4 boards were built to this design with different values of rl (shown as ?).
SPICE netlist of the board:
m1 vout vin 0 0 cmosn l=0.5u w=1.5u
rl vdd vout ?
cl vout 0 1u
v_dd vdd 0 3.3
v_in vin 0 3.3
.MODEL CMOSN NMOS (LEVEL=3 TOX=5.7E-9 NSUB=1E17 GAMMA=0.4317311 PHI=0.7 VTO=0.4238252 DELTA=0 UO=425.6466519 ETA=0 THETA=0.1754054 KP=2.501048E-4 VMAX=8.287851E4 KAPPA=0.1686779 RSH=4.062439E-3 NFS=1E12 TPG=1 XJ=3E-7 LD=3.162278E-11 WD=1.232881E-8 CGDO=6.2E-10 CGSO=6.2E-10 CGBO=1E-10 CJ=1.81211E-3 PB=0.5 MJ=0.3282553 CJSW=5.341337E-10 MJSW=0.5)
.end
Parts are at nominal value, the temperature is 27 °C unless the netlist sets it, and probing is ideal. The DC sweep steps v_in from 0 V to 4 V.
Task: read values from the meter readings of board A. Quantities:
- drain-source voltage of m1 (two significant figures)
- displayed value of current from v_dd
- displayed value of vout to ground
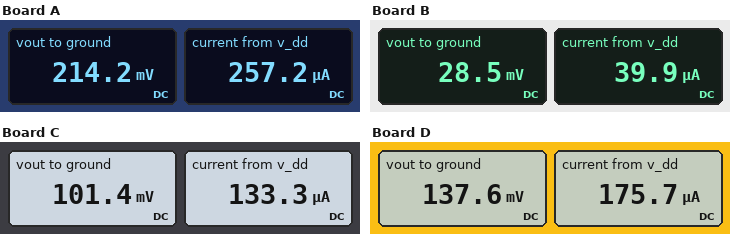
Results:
210 mV
257.2 µA
214.2 mV
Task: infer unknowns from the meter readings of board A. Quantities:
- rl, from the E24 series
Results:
12 kΩ
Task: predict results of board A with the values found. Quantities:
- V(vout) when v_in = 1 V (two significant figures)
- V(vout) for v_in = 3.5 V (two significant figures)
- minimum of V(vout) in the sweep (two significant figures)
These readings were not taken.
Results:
2.2 V
200 mV
180 mV
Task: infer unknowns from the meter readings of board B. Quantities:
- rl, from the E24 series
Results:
82 kΩ
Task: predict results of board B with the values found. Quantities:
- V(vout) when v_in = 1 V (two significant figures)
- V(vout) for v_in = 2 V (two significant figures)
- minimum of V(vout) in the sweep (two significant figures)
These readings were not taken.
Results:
110 mV
44 mV
25 mV
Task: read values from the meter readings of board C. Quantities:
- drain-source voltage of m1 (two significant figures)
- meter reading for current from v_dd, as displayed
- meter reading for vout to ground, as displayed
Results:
100 mV
133.3 µA
101.4 mV
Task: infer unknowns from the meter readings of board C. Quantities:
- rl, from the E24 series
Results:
24 kΩ
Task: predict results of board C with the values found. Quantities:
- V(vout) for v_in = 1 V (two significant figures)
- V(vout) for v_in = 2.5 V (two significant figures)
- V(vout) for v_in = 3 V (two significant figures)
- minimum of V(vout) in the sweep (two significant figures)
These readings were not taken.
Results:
1.2 V
130 mV
110 mV
87 mV
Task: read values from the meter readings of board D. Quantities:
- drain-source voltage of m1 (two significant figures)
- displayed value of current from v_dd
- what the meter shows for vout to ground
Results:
140 mV
175.7 µA
137.6 mV
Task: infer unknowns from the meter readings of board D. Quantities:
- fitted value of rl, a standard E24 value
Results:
18 kΩ
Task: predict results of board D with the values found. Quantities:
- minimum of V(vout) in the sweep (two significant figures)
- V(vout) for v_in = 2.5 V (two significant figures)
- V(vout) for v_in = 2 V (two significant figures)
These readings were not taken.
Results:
120 mV
180 mV
230 mV
